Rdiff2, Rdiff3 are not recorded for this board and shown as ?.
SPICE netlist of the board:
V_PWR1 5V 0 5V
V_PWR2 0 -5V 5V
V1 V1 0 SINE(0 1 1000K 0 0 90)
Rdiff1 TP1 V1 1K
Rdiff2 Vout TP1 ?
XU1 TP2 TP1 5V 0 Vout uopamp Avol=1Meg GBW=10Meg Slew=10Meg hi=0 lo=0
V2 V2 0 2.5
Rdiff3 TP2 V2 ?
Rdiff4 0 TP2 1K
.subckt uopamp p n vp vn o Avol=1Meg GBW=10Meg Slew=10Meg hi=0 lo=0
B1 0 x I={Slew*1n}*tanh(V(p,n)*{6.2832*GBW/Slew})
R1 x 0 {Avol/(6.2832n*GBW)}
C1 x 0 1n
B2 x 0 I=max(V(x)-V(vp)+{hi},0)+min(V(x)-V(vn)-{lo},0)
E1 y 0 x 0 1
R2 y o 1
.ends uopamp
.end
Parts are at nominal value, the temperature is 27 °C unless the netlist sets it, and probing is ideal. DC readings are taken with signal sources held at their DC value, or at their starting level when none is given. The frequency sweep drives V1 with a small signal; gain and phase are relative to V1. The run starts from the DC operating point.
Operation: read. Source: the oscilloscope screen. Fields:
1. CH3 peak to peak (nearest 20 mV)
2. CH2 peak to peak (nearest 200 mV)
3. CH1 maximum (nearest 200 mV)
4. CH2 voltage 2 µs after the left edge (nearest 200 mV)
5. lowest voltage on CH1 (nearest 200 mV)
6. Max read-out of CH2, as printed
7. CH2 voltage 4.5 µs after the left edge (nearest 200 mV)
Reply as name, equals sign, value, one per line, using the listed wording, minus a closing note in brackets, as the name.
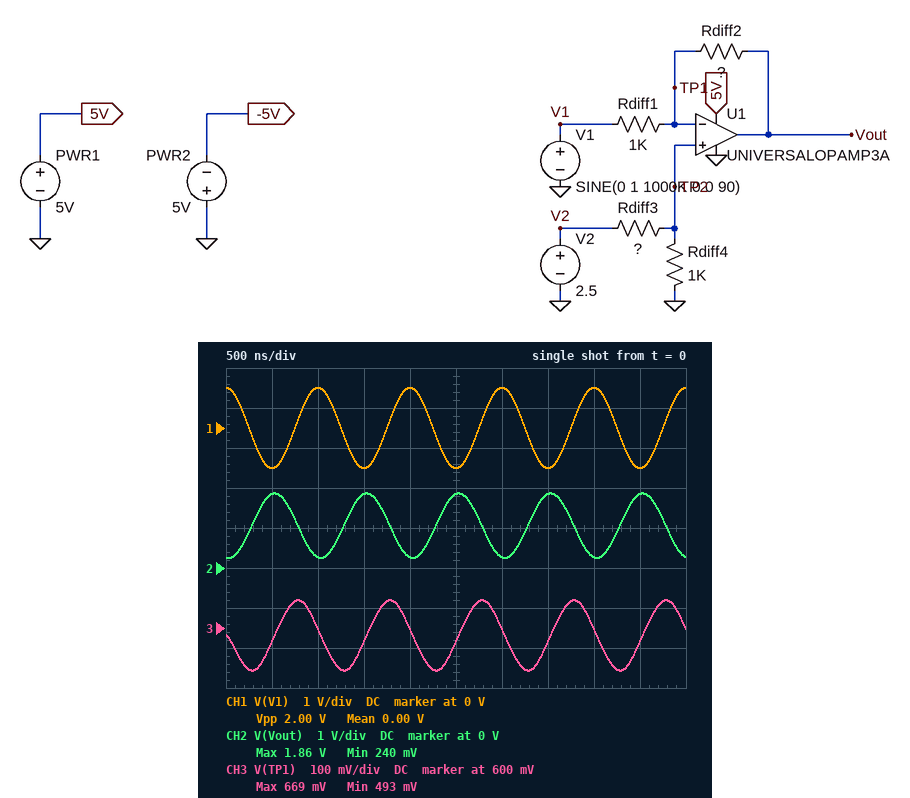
CH3 peak to peak = 180 mV
CH2 peak to peak = 1.6 V
CH1 maximum = 1.0 V
CH2 voltage 2 µs after the left edge = 200 mV
lowest voltage on CH1 = -1.0 V
Max read-out of CH2, as printed = 1.86 V
CH2 voltage 4.5 µs after the left edge = 1.8 V
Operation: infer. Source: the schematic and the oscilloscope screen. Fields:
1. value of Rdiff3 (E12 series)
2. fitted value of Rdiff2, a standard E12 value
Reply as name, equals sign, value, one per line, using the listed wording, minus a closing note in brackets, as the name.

value of Rdiff3 = 3.3 kΩ
fitted value of Rdiff2, a standard E12 value = 820 Ω
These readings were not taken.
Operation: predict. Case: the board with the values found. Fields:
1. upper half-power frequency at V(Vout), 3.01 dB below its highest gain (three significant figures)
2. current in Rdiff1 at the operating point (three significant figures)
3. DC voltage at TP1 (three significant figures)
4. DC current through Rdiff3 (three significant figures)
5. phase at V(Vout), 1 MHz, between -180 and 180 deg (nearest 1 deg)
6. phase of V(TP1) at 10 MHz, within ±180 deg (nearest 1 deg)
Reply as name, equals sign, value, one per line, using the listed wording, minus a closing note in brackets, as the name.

upper half-power frequency at V(Vout), 3.01 dB below its highest gain = 5.49 MHz
current in Rdiff1 at the operating point = 419 µA
DC voltage at TP1 = 581 mV
DC current through Rdiff3 = 581 µA
phase at V(Vout), 1 MHz, between -180 and 180 deg = 170 deg
phase of V(TP1) at 10 MHz, within ±180 deg = 29 deg
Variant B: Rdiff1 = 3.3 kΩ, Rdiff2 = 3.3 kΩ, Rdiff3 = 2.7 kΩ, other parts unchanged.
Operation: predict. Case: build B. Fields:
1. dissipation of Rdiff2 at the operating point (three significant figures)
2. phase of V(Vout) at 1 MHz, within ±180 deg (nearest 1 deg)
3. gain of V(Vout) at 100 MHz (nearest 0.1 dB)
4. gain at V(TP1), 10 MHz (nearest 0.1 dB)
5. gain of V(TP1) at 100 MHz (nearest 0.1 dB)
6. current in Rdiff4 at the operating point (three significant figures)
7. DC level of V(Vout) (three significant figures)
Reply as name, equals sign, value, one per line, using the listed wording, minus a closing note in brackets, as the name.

dissipation of Rdiff2 at the operating point = 31.9 µW
phase of V(Vout) at 1 MHz, within ±180 deg = 169 deg
gain of V(Vout) at 100 MHz = -26.0 dB
gain at V(TP1), 10 MHz = -7.0 dB
gain of V(TP1) at 100 MHz = -6.0 dB
current in Rdiff4 at the operating point = 676 µA
DC level of V(Vout) = 351 mV
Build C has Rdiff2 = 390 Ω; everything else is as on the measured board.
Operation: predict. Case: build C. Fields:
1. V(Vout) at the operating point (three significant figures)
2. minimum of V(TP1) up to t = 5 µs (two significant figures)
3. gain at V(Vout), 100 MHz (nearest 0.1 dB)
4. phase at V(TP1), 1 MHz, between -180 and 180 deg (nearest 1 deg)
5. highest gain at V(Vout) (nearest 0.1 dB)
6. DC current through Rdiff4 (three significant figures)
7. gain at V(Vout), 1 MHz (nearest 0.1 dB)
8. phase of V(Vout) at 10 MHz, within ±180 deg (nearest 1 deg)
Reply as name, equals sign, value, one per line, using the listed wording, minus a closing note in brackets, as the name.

V(Vout) at the operating point = 418 mV
minimum of V(TP1) up to t = 5 µs = 540 mV
gain at V(Vout), 100 MHz = -31.1 dB
phase at V(TP1), 1 MHz, between -180 and 180 deg = 82 deg
highest gain at V(Vout) = -8.2 dB
DC current through Rdiff4 = 581 µA
gain at V(Vout), 1 MHz = -8.3 dB
phase of V(Vout) at 10 MHz, within ±180 deg = 126 deg
